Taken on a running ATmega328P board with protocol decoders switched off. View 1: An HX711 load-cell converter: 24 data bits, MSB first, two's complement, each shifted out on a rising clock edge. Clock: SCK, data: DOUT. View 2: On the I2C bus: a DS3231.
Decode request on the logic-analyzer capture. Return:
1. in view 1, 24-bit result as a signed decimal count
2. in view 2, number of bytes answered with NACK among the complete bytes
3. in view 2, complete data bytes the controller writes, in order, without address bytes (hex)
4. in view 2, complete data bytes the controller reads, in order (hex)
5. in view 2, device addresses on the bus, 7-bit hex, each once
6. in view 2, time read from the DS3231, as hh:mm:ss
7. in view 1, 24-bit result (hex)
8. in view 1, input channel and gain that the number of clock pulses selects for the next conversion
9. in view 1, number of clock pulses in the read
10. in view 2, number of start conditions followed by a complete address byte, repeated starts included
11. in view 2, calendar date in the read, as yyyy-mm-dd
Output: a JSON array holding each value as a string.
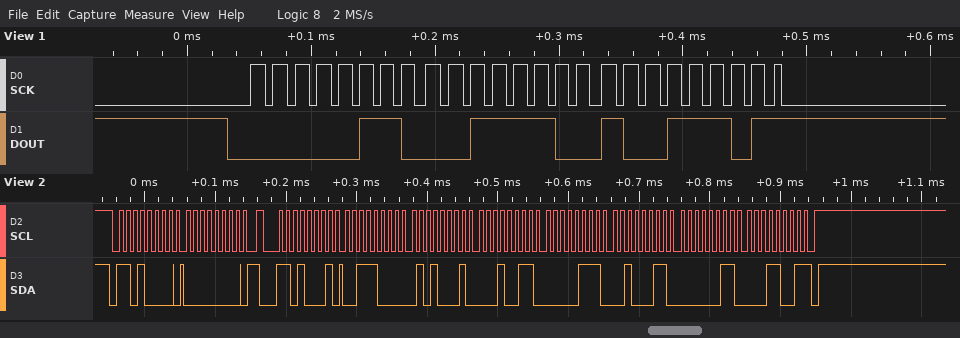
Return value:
["408733", "1", "00", "38 51 13 07 23 03 19", "0x68", "13:51:38", "0x063C9D", "channel A, gain 128", "25", "2", "2019-03-23"]
